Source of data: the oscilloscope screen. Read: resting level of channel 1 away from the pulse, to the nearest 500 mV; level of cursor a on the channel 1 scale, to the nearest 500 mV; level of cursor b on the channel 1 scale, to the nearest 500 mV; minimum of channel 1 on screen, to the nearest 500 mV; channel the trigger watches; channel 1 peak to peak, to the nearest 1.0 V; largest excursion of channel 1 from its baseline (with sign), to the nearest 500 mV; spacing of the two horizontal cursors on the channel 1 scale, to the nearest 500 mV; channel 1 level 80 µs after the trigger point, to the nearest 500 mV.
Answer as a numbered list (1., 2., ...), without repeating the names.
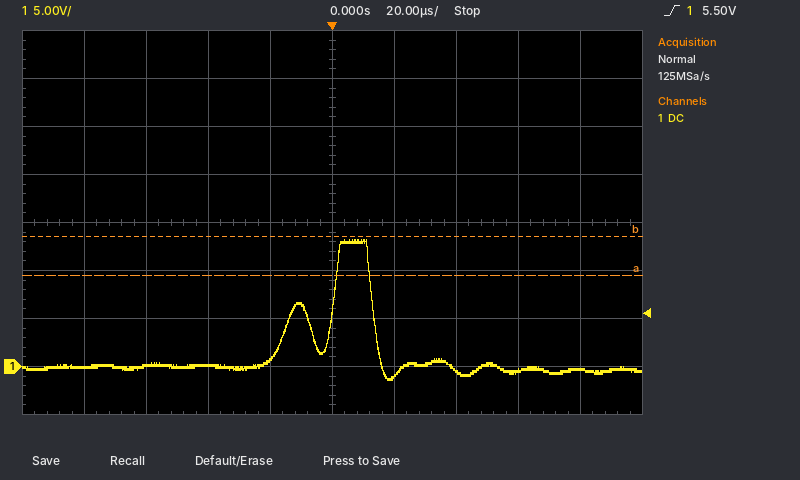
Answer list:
1. 0.0 V
2. 9.5 V
3. 13.5 V
4. -1.5 V
5. channel 1
6. 15.0 V
7. +13.5 V
8. 4.0 V
9. -500 mV
